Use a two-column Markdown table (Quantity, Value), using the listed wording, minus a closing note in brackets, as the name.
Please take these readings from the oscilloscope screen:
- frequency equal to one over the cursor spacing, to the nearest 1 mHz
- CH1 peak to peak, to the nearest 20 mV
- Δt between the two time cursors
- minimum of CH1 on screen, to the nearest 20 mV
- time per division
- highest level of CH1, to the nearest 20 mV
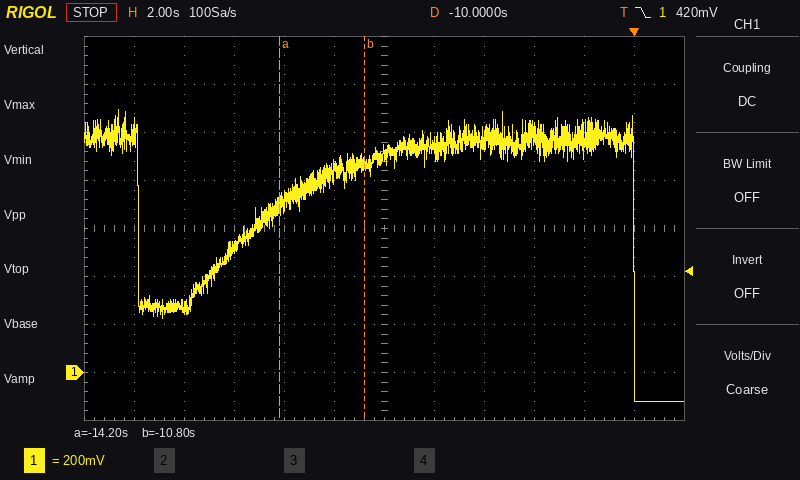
| Quantity | Value |
|---|---|
| frequency equal to one over the cursor spacing, to the nearest 1 mHz | 294 mHz |
| CH1 peak to peak, to the nearest 20 mV | 1.22 V |
| Δt between the two time cursors | 3.4 s |
| minimum of CH1 on screen, to the nearest 20 mV | -120 mV |
| time per division | 2 s |
| highest level of CH1, to the nearest 20 mV | 1.10 V |
